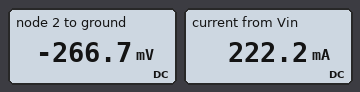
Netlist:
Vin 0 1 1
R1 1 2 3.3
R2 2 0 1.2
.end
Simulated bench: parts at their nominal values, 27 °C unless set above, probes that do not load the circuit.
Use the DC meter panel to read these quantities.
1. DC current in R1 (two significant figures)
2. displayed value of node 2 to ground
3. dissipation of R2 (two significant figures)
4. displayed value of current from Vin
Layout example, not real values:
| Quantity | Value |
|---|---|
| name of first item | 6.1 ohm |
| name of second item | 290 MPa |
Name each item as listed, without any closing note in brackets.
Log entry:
| Quantity | Value |
|---|---|
| DC current in R1 | 220 mA |
| displayed value of node 2 to ground | -266.7 mV |
| dissipation of R2 | 59 mW |
| displayed value of current from Vin | 222.2 mA |
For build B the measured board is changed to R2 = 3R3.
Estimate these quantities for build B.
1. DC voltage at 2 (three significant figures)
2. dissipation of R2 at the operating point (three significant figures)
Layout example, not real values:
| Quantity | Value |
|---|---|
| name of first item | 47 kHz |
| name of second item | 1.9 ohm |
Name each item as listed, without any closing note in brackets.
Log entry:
| Quantity | Value |
|---|---|
| DC voltage at 2 | -500 mV |
| dissipation of R2 at the operating point | 75.8 mW |
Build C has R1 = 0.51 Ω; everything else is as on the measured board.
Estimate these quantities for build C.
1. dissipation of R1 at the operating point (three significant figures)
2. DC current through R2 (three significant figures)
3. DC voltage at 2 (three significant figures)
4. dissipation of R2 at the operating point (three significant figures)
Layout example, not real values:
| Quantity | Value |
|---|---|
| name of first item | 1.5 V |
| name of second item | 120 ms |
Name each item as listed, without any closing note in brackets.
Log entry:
| Quantity | Value |
|---|---|
| dissipation of R1 at the operating point | 174 mW |
| DC current through R2 | 585 mA |
| DC voltage at 2 | -702 mV |
| dissipation of R2 at the operating point | 410 mW |
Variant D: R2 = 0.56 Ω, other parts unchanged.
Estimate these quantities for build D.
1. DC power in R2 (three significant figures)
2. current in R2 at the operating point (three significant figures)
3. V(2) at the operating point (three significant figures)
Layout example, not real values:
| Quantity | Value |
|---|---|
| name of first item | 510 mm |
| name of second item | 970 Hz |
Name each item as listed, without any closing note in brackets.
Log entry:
| Quantity | Value |
|---|---|
| DC power in R2 | 37.6 mW |
| current in R2 at the operating point | 259 mA |
| V(2) at the operating point | -145 mV |
